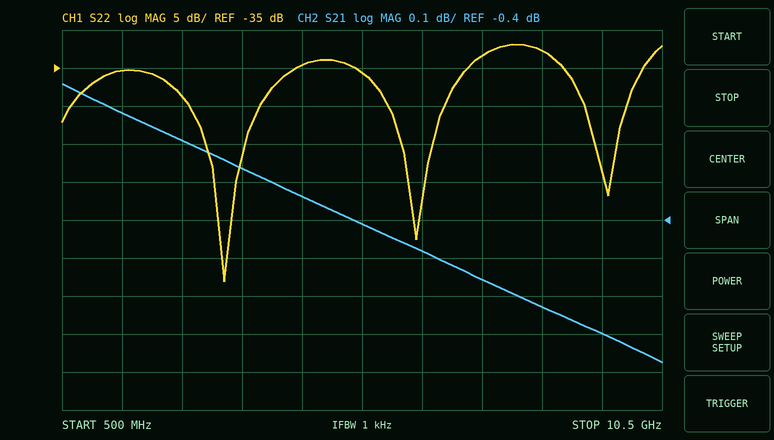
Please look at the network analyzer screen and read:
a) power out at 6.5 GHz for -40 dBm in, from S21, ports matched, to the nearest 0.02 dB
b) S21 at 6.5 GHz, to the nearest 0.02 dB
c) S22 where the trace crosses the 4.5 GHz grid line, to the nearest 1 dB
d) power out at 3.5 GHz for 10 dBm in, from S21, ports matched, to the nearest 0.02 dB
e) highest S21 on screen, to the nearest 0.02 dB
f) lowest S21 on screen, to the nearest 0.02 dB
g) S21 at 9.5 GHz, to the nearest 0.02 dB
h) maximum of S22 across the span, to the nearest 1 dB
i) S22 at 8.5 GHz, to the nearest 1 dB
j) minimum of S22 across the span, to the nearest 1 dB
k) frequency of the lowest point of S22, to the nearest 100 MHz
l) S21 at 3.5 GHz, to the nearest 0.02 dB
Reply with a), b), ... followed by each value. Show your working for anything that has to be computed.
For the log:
a) -40 dBm + (-0.48 dB) = -40.48 dBm
b) -0.48 dB
c) -35 dB
d) 10 dBm + (-0.26 dB) = 9.74 dBm
e) -0.04 dB
f) -0.78 dB
g) -0.70 dB
h) -32 dB
i) -33 dB
j) -63 dB
k) 3.2 GHz
l) -0.26 dB
